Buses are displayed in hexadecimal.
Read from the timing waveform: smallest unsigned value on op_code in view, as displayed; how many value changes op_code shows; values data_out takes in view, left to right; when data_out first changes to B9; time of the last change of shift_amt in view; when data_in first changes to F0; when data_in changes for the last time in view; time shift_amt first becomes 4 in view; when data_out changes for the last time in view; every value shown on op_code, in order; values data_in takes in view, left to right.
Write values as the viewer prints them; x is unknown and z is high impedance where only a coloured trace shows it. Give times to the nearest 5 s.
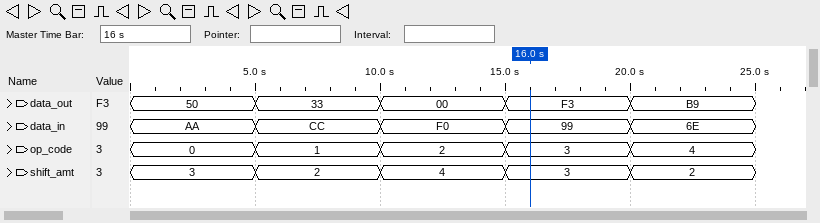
0
4
50, 33, 00, F3, B9
20 s
20 s
10 s
20 s
10 s
20 s
0, 1, 2, 3, 4
AA, CC, F0, 99, 6E
